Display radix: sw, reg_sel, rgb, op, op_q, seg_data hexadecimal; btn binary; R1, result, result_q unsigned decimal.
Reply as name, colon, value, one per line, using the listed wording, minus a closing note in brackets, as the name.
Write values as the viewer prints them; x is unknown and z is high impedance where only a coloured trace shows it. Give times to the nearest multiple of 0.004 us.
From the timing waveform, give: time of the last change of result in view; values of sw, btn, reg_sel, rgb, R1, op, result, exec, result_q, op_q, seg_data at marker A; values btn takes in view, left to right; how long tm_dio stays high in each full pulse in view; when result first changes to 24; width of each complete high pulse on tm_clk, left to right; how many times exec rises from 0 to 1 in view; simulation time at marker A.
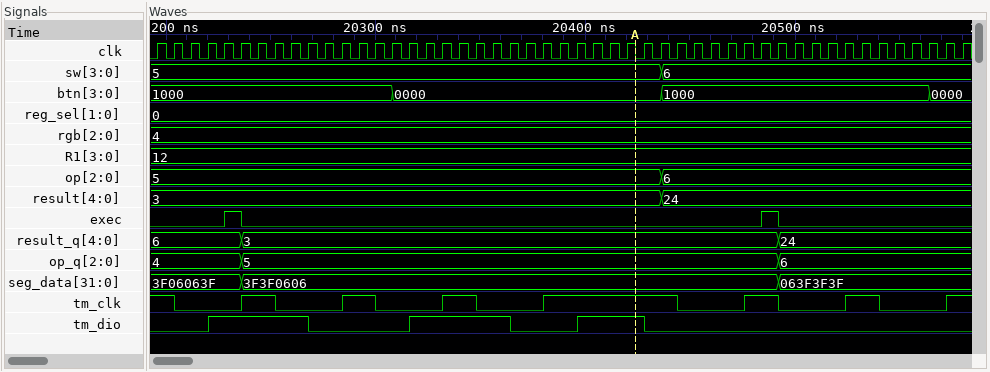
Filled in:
time of the last change of result in view: 20.436 us
values of sw, btn, reg_sel, rgb, R1, op, result, exec, result_q, op_q, seg_data at marker A: sw=5, btn=0000, reg_sel=0, rgb=4, R1=12, op=5, result=3, exec=0, result_q=3, op_q=5, seg_data=3F3F0606
values btn takes in view, left to right: 1000, 0000, 1000, 0000
how long tm_dio stays high in each full pulse in view: 0.048 us, 0.048 us, 0.032 us
when result first changes to 24: 20.436 us
width of each complete high pulse on tm_clk, left to right: 0.016 us, 0.016 us, 0.016 us, 0.064 us, 0.016 us, 0.016 us
how many times exec rises from 0 to 1 in view: 2
simulation time at marker A: 20.424 us
